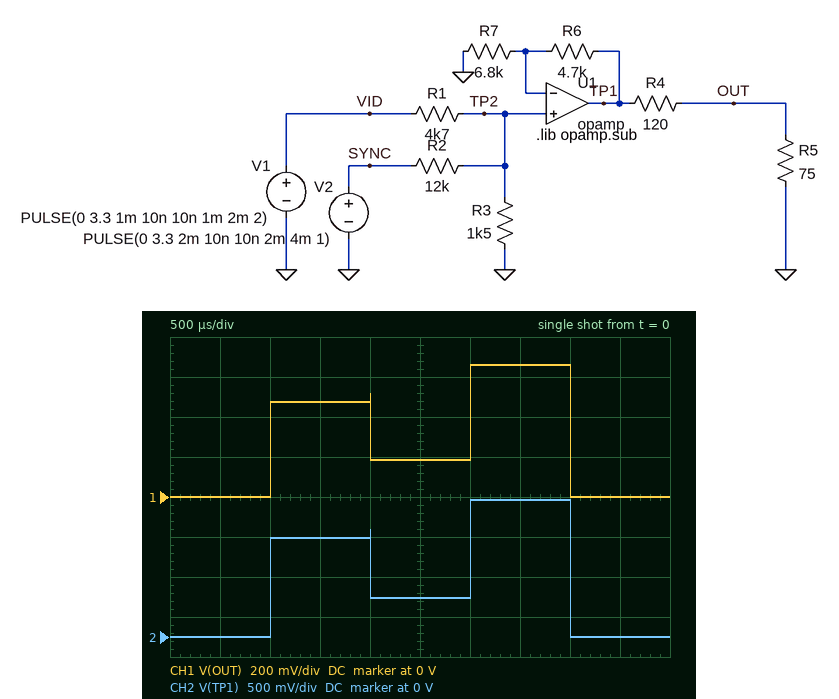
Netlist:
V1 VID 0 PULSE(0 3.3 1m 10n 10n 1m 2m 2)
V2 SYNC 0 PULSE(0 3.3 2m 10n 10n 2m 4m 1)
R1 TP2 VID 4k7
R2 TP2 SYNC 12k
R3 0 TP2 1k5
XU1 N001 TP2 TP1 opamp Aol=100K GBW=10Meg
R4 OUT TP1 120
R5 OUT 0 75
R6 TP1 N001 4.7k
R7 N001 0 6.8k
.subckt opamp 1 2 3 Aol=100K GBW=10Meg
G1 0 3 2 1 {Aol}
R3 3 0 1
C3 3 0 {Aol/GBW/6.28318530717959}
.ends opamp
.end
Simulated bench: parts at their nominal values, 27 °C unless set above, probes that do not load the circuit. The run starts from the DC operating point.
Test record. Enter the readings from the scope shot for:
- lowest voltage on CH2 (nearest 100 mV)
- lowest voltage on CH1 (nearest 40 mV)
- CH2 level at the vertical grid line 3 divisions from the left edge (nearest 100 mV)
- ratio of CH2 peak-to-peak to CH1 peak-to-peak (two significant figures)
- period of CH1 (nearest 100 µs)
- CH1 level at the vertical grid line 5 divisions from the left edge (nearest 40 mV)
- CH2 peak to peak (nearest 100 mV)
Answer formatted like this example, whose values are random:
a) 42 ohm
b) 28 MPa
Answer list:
a) 0 V
b) 0 V
c) 1.2 V
d) 2.6
e) 2.0 ms
f) 200 mV
g) 1.7 V
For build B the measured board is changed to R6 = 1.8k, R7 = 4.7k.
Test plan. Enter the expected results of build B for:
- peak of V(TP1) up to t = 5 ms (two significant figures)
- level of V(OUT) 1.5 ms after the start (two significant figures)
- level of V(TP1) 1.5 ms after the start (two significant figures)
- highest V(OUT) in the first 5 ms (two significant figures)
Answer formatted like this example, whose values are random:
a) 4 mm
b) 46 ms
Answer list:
a) 1.4 V
b) 390 mV
c) 1.0 V
d) 540 mV
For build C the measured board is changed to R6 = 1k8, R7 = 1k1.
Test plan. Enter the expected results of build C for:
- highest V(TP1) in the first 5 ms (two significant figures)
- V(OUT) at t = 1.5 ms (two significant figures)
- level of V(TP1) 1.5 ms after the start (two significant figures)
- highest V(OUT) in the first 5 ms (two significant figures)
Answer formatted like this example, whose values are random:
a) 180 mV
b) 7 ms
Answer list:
a) 2.7 V
b) 740 mV
c) 1.9 V
d) 1.0 V
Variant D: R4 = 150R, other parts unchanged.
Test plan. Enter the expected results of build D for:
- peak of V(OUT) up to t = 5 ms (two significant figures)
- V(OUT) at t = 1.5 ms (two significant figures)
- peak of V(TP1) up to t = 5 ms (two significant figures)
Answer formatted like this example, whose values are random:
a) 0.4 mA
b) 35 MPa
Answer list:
a) 570 mV
b) 410 mV
c) 1.7 V
